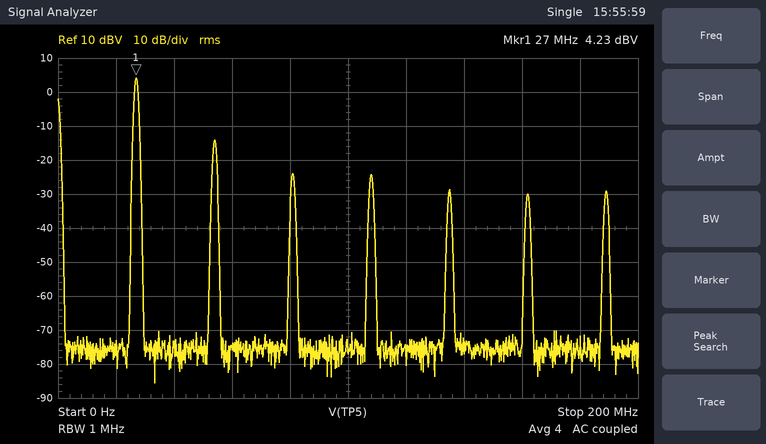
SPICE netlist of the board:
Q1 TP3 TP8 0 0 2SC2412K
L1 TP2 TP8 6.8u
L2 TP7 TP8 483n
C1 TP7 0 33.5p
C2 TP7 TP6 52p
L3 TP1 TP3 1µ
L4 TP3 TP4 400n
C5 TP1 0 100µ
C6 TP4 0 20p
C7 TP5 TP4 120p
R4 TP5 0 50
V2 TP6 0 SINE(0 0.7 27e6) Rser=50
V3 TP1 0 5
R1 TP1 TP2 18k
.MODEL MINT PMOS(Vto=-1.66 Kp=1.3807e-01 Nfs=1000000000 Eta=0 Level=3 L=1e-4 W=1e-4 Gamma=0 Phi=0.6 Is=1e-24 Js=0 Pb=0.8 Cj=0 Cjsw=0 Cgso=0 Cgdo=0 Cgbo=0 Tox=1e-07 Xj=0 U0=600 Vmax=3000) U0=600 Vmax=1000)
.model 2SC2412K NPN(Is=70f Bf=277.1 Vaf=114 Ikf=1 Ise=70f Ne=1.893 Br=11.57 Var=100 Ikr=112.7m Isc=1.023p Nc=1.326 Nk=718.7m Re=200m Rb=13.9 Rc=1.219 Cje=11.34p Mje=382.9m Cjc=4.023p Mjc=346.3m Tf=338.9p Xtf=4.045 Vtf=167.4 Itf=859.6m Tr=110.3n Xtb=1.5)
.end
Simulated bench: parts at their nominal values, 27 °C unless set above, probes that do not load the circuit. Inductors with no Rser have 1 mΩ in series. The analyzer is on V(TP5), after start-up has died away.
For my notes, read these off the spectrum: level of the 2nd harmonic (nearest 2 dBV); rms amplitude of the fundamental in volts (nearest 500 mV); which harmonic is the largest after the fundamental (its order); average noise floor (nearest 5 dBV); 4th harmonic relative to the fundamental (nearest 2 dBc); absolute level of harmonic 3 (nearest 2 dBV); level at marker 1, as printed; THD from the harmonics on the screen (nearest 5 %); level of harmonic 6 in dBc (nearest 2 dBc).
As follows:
-14 dBV
1.5 V
2
-75 dBV
-28 dBc
-24 dBV
4.23 dBV
15 %
-34 dBc
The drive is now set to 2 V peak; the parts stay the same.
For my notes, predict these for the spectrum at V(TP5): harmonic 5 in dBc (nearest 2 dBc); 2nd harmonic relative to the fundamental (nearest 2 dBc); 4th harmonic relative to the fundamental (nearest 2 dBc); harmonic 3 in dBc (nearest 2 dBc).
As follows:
-26 dBc
-6 dBc
-22 dBc
-26 dBc
